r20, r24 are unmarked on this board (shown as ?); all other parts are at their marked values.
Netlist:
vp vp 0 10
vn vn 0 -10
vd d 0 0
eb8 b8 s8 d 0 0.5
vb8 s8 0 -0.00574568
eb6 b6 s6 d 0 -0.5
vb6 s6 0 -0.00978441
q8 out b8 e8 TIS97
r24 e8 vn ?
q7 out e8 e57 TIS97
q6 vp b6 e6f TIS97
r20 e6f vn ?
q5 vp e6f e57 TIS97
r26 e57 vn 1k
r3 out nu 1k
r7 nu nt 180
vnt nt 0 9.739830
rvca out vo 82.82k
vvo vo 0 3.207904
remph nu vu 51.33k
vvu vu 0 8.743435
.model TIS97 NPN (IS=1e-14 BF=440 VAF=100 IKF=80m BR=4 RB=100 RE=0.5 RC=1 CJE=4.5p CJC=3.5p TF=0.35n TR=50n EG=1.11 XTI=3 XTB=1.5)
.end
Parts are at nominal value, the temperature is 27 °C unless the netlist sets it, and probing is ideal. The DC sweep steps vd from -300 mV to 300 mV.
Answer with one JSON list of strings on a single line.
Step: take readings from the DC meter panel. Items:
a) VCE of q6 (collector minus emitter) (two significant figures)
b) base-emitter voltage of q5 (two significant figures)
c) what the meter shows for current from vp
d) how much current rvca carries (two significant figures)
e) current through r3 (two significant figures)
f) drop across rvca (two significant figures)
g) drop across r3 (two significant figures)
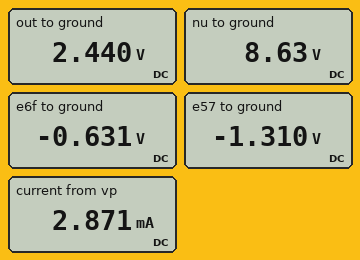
["11 V", "680 mV", "2.871 mA", "9.3 µA", "6.2 mA", "770 mV", "6.2 V"]
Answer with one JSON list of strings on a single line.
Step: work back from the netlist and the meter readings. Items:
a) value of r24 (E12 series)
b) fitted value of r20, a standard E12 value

["100 kΩ", "33 kΩ"]
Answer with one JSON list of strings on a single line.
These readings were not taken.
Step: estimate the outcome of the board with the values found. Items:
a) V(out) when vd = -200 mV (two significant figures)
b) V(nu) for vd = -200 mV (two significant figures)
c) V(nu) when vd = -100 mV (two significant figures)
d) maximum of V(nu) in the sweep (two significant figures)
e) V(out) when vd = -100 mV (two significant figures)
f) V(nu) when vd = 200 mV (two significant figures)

["9.5 V", "9.7 V", "9.6 V", "9.7 V", "8.6 V", "8.2 V"]
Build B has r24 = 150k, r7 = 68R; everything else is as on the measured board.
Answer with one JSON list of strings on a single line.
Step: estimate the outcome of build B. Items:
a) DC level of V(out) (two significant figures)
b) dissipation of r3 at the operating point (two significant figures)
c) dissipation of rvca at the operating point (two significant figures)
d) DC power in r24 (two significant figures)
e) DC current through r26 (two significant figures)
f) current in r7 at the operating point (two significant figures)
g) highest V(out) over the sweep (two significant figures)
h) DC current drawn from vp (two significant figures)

["2.6 V", "44 mW", "4.0 µW", "590 µW", "8.7 mA", "6.7 mA", "9.6 V", "2.4 mA"]
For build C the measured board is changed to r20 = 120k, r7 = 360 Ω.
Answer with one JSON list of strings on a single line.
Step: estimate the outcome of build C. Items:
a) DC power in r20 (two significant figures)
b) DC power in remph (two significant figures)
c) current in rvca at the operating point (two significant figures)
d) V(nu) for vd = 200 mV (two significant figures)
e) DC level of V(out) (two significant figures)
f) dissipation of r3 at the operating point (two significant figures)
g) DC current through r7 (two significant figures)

["740 µW", "5.3 µW", "9.4 µA", "7.0 V", "4.0 V", "18 mW", "4.2 mA"]
